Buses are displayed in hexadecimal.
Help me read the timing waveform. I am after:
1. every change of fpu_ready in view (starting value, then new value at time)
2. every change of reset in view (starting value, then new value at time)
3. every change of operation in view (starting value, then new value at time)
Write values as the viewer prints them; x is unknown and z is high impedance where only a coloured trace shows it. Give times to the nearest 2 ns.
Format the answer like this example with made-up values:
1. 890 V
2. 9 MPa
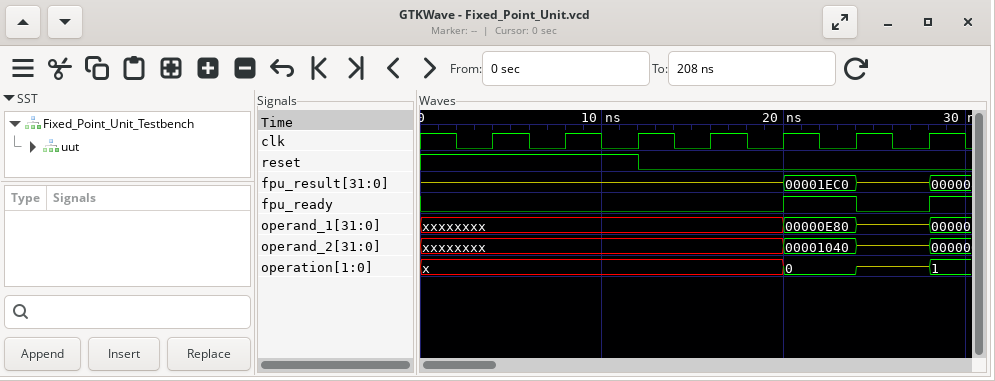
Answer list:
1. 0, 1 at 20 ns, 0 at 24 ns, 1 at 28 ns
2. 1, 0 at 12 ns
3. x, 0 at 20 ns, z at 24 ns, 1 at 28 ns
